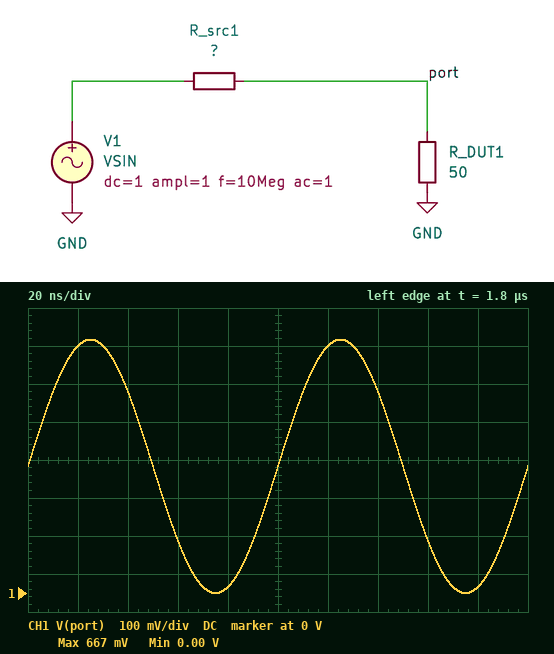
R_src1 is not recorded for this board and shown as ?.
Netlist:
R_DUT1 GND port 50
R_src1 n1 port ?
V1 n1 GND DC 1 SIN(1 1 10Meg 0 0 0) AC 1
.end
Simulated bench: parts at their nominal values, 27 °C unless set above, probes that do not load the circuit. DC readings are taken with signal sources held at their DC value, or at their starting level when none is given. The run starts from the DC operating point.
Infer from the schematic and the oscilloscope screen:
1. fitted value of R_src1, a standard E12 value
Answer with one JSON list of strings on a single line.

["100 Ω"]
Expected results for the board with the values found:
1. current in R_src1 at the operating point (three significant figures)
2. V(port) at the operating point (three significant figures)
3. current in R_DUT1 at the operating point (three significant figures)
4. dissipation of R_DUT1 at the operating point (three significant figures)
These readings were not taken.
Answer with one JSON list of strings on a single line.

["6.67 mA", "333 mV", "6.67 mA", "2.22 mW"]
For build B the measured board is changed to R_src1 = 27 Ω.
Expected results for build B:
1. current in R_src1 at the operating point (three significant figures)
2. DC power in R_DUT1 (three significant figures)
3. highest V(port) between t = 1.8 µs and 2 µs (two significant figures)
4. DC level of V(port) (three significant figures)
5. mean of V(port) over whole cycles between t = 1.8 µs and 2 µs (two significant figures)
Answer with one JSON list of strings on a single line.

["13.0 mA", "8.43 mW", "1.3 V", "649 mV", "650 mV"]
